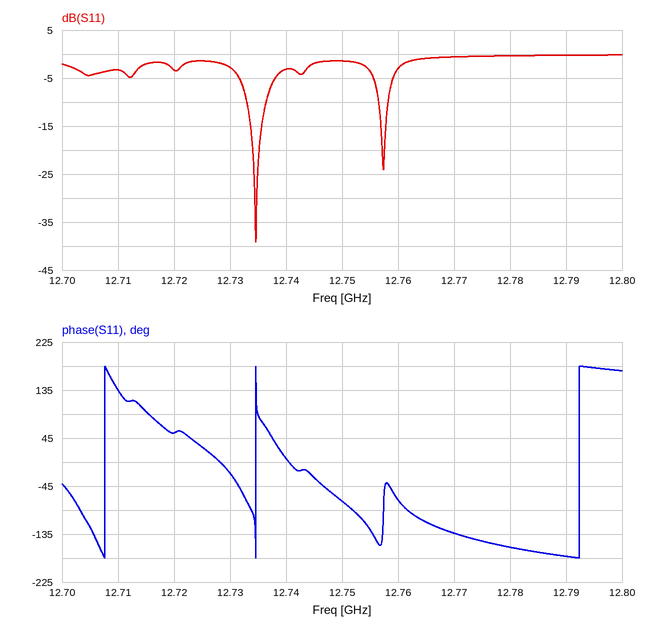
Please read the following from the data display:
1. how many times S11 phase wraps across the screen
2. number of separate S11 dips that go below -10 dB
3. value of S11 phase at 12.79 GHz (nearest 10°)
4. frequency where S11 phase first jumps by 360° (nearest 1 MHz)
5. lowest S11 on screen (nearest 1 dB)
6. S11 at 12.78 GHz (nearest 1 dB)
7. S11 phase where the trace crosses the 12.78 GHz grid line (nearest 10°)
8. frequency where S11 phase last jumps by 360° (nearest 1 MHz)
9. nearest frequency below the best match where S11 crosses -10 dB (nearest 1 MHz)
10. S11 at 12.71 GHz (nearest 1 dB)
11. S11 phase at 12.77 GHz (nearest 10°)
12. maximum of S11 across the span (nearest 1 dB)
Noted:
3
2
-180°
12.708 GHz
-39 dB
0 dB
-160°
12.792 GHz
12.733 GHz
-3 dB
-130°
0 dB
